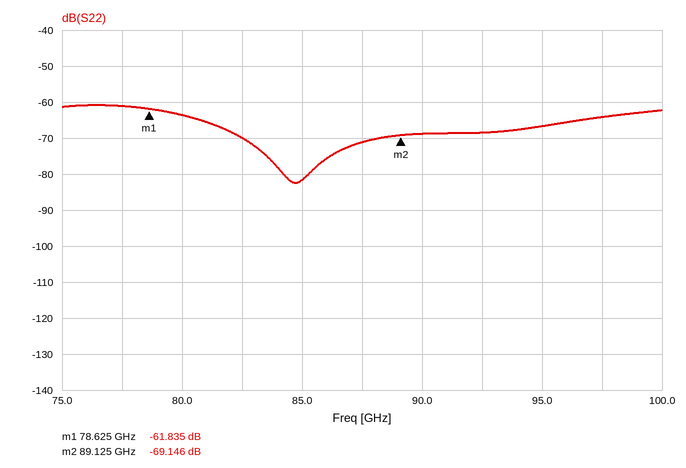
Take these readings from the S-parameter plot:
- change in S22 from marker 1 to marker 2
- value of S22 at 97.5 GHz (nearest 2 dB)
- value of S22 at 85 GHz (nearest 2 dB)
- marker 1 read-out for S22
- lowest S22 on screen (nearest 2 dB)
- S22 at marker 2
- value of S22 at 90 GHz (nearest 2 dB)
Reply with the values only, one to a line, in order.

-7.311 dB
-64 dB
-82 dB
-61.835 dB
-82 dB
-69.146 dB
-68 dB
